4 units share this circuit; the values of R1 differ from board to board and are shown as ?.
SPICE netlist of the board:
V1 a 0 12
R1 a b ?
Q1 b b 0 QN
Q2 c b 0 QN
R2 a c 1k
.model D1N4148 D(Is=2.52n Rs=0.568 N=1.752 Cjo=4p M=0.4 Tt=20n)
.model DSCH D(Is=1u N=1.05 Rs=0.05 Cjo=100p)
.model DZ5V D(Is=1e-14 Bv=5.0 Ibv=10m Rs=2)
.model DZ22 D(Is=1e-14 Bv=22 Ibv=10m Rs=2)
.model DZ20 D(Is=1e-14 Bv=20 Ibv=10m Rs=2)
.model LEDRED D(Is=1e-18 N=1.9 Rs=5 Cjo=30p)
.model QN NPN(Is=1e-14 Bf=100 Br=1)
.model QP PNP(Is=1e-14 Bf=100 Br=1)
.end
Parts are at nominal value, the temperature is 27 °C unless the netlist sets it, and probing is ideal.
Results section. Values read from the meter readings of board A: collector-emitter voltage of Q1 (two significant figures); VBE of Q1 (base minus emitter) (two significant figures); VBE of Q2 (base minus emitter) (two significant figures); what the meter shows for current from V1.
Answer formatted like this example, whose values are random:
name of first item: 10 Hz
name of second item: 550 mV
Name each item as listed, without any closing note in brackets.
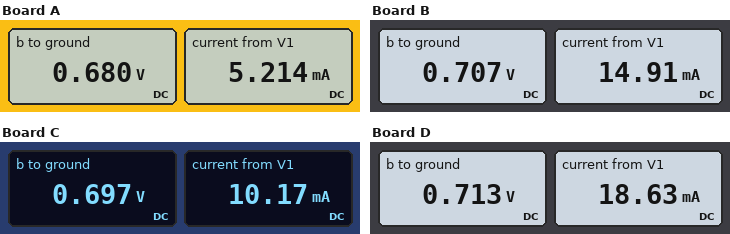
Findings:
collector-emitter voltage of Q1: 680 mV
VBE of Q1 (base minus emitter): 680 mV
VBE of Q2 (base minus emitter): 680 mV
what the meter shows for current from V1: 5.214 mA
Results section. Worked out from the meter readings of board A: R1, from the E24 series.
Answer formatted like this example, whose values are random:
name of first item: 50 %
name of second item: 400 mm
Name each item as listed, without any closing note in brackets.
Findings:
R1, from the E24 series: 4.3 kΩ
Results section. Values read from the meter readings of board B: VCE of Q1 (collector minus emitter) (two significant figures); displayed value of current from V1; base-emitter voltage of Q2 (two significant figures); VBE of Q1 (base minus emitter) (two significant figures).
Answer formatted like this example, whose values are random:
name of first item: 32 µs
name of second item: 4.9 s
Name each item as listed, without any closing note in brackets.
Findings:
VCE of Q1 (collector minus emitter): 710 mV
displayed value of current from V1: 14.91 mA
base-emitter voltage of Q2: 710 mV
VBE of Q1 (base minus emitter): 710 mV
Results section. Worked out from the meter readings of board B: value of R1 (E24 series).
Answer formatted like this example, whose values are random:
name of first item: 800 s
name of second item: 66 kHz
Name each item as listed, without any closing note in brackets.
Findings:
value of R1: 1.5 kΩ
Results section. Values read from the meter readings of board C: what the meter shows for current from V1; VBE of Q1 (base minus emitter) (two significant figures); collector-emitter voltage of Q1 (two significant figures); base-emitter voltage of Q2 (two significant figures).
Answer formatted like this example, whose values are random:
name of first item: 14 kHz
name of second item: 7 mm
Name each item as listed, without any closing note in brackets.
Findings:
what the meter shows for current from V1: 10.17 mA
VBE of Q1 (base minus emitter): 700 mV
collector-emitter voltage of Q1: 700 mV
base-emitter voltage of Q2: 700 mV
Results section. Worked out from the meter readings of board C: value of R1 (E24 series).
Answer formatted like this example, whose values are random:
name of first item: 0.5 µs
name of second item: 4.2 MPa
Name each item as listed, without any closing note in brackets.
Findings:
value of R1: 2.2 kΩ
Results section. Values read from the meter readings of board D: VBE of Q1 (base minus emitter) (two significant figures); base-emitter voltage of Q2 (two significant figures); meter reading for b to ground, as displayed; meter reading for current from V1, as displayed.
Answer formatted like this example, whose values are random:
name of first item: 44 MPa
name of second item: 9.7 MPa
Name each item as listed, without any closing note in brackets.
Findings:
VBE of Q1 (base minus emitter): 710 mV
base-emitter voltage of Q2: 710 mV
meter reading for b to ground, as displayed: 0.713 V
meter reading for current from V1, as displayed: 18.63 mA
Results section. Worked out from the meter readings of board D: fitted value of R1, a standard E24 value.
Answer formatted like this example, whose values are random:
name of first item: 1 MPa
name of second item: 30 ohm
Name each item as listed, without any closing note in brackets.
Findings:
fitted value of R1, a standard E24 value: 1.2 kΩ
